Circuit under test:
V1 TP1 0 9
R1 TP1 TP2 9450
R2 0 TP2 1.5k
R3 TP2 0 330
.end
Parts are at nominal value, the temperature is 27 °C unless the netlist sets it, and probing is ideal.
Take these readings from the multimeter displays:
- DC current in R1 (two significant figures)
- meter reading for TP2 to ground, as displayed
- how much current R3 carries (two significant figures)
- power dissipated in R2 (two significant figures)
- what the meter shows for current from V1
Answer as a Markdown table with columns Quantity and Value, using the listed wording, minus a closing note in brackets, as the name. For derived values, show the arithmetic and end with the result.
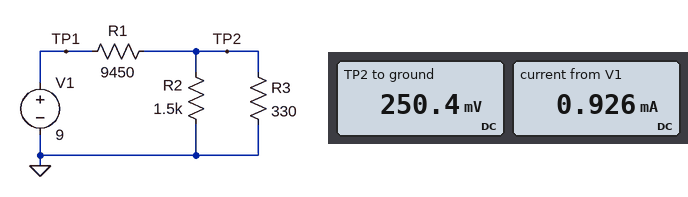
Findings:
| Quantity | Value |
|---|---|
| DC current in R1 | (9 V - 250.4 mV) / 9.45 kΩ = 930 µA |
| meter reading for TP2 to ground, as displayed | 250.4 mV |
| how much current R3 carries | (250.4 mV) / 330 Ω = 760 µA |
| power dissipated in R2 | (250.4 mV)^2 / 1.5 kΩ = 42 µW |
| what the meter shows for current from V1 | 0.926 mA |
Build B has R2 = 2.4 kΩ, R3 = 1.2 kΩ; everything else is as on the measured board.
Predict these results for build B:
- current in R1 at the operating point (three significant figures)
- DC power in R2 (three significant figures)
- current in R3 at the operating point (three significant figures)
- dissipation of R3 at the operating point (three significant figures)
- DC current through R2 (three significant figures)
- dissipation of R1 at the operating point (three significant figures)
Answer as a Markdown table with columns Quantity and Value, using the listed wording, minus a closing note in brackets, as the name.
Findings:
| Quantity | Value |
|---|---|
| current in R1 at the operating point | 878 µA |
| DC power in R2 | 206 µW |
| current in R3 at the operating point | 585 µA |
| dissipation of R3 at the operating point | 411 µW |
| DC current through R2 | 293 µA |
| dissipation of R1 at the operating point | 7.29 mW |
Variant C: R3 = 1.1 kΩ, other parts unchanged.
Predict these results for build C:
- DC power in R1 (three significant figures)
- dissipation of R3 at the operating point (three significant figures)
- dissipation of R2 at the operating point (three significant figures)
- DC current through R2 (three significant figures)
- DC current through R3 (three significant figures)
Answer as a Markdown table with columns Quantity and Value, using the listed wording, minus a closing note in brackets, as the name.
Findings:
| Quantity | Value |
|---|---|
| DC power in R1 | 7.53 mW |
| dissipation of R3 at the operating point | 292 µW |
| dissipation of R2 at the operating point | 214 µW |
| DC current through R2 | 378 µA |
| DC current through R3 | 515 µA |
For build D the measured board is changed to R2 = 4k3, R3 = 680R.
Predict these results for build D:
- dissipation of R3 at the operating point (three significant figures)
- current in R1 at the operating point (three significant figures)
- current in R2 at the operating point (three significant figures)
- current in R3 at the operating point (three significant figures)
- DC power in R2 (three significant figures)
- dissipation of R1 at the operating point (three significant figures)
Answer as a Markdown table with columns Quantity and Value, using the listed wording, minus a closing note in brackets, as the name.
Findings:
| Quantity | Value |
|---|---|
| dissipation of R3 at the operating point | 408 µW |
| current in R1 at the operating point | 897 µA |
| current in R2 at the operating point | 122 µA |
| current in R3 at the operating point | 774 µA |
| DC power in R2 | 64.5 µW |
| dissipation of R1 at the operating point | 7.60 mW |
